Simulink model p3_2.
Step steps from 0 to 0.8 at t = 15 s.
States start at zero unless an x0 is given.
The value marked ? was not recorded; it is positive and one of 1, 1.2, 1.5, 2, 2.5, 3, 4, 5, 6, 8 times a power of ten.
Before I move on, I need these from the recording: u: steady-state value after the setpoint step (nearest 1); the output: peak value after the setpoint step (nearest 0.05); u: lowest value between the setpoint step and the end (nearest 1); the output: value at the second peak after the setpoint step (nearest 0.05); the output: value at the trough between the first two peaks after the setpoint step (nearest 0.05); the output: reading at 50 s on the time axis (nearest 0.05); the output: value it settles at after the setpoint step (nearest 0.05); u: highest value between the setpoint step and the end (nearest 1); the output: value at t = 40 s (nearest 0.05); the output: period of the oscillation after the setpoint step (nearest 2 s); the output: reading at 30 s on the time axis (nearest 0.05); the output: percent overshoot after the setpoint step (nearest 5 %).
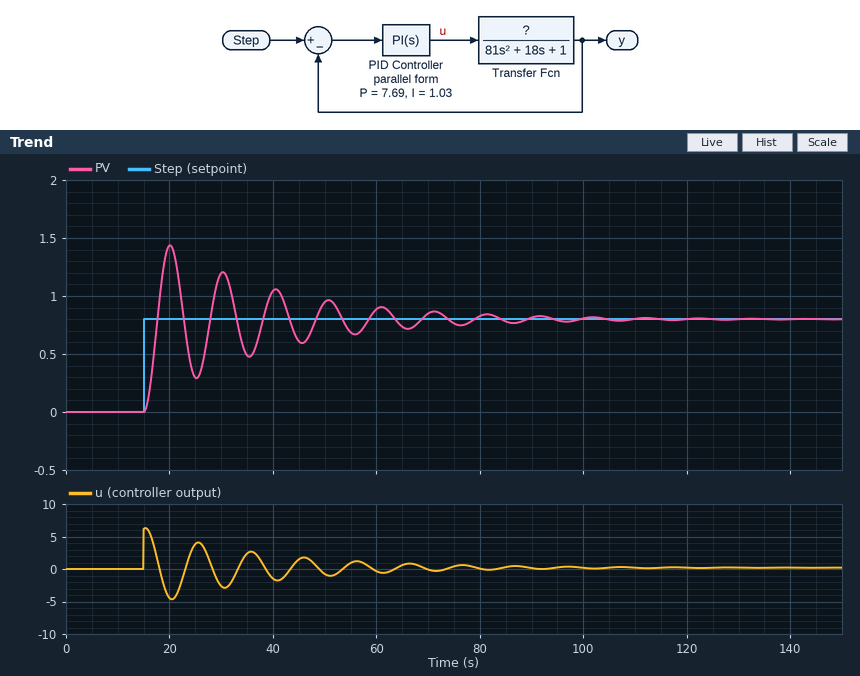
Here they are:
0
1.45
-5
1.20
0.30
0.95
0.80
6
1.05
10 s
1.20
80 %
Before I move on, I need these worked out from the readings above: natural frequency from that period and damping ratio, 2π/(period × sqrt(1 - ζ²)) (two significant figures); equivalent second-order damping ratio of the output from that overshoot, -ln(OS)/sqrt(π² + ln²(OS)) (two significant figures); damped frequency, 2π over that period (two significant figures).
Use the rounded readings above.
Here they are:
0.63 rad/s
0.071
0.63 rad/s
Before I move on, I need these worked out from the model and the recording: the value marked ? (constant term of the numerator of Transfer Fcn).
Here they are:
4
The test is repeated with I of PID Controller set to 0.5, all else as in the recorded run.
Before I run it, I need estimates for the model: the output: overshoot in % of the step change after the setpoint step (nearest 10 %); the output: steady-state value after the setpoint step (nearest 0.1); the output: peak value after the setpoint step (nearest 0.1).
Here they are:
70 %
0.8
1.3
